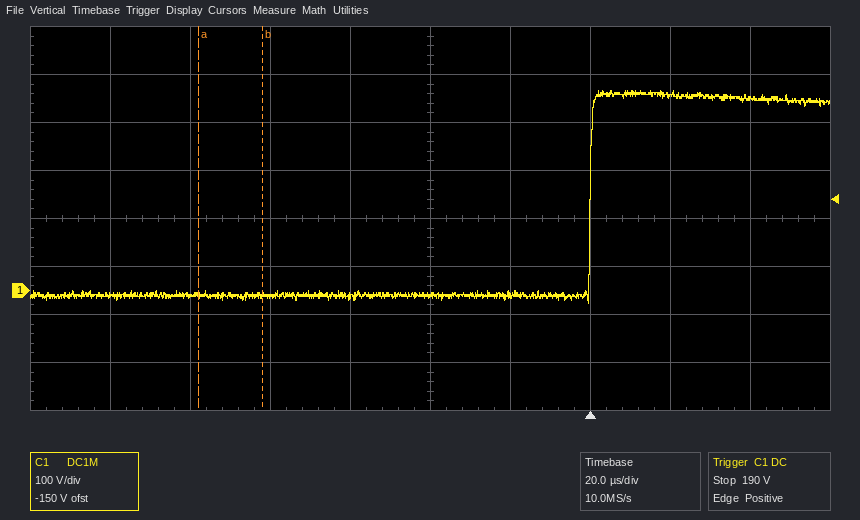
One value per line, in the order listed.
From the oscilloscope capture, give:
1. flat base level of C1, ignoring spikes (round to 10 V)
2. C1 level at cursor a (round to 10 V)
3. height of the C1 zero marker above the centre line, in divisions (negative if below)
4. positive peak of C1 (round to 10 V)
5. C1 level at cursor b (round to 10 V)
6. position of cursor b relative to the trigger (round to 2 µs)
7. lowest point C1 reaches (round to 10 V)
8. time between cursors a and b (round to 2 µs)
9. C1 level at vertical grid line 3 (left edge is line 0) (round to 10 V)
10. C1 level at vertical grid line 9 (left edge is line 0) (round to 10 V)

-10 V
-10 V
-1.5 div
420 V
-10 V
-82 µs
-30 V
16 µs
-10 V
400 V
